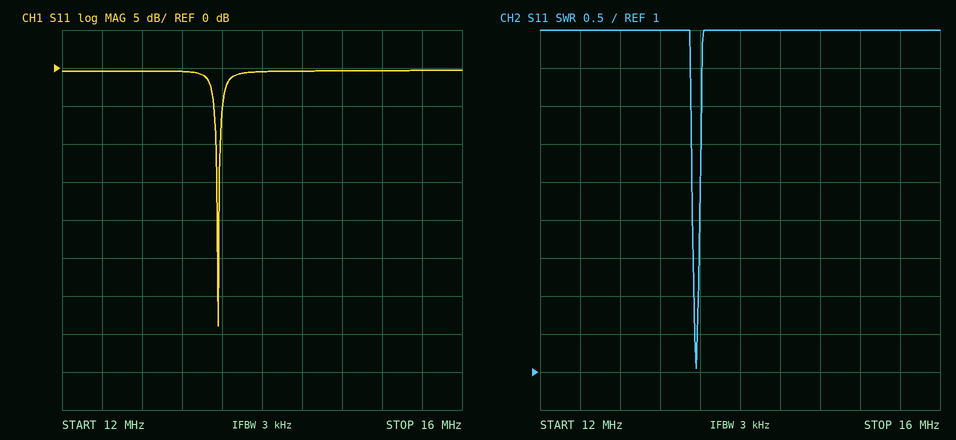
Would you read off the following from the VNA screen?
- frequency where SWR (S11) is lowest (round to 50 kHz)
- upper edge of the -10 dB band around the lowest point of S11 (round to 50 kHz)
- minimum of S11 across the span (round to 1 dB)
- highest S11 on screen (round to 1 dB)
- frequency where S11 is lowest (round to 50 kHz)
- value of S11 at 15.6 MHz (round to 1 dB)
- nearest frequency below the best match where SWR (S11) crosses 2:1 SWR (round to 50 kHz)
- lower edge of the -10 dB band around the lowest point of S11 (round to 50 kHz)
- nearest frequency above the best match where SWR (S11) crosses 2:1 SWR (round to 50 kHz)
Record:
13.55 MHz
13.60 MHz
-34 dB
0 dB
13.55 MHz
0 dB
13.55 MHz
13.55 MHz
13.60 MHz
